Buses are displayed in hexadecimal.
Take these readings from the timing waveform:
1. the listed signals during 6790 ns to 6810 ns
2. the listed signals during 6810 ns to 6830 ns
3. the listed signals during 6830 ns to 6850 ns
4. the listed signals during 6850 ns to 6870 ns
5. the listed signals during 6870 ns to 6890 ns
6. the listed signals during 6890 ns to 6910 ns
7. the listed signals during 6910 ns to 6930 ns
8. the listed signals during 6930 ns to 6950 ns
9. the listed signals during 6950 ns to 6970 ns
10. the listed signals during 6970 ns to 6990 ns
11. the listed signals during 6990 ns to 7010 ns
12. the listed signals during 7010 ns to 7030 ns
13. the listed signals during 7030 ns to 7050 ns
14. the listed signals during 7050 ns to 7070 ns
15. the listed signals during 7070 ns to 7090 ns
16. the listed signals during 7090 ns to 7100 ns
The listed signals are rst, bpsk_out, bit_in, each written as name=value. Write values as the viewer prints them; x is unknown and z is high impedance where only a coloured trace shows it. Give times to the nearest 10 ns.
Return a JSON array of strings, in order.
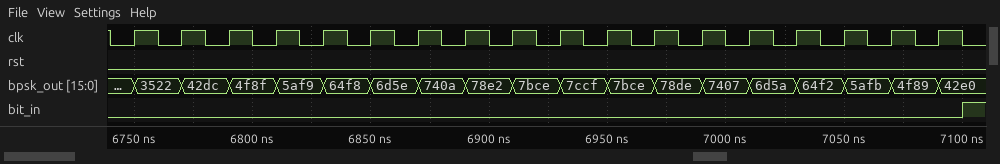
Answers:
["rst=0, bpsk_out=4f8f, bit_in=0", "rst=0, bpsk_out=5af9, bit_in=0", "rst=0, bpsk_out=64f8, bit_in=0", "rst=0, bpsk_out=6d5e, bit_in=0", "rst=0, bpsk_out=740a, bit_in=0", "rst=0, bpsk_out=78e2, bit_in=0", "rst=0, bpsk_out=7bce, bit_in=0", "rst=0, bpsk_out=7ccf, bit_in=0", "rst=0, bpsk_out=7bce, bit_in=0", "rst=0, bpsk_out=78de, bit_in=0", "rst=0, bpsk_out=7407, bit_in=0", "rst=0, bpsk_out=6d5a, bit_in=0", "rst=0, bpsk_out=64f2, bit_in=0", "rst=0, bpsk_out=5afb, bit_in=0", "rst=0, bpsk_out=4f89, bit_in=0", "rst=0, bpsk_out=42e0, bit_in=0"]
